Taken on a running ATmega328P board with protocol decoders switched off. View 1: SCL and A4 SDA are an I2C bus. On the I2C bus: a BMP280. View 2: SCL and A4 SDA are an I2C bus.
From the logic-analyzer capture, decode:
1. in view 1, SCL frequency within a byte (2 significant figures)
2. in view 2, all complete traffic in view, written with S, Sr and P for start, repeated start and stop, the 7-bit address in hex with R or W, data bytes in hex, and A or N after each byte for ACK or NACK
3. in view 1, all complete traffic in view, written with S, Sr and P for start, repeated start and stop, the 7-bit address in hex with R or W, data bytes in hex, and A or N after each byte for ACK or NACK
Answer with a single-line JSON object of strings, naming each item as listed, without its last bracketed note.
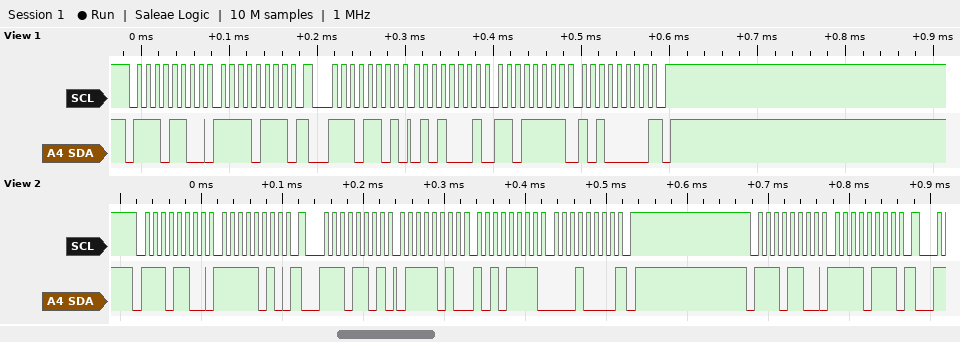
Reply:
{"in view 1, SCL frequency within a byte": "100 kHz", "in view 2, all complete traffic in view, written with S, Sr and P for start, repeated start and stop, the 7-bit address in hex with R or W, data bytes in hex, and A or N after each byte for ACK or NACK": "S 76W A FA A Sr 76R A 7A A AF A 10 N P S 76W A F7 A", "in view 1, all complete traffic in view, written with S, Sr and P for start, repeated start and stop, the 7-bit address in hex with R or W, data bytes in hex, and A or N after each byte for ACK or NACK": "S 76W A F7 A Sr 76R A 51 A DF A A0 N P"}
